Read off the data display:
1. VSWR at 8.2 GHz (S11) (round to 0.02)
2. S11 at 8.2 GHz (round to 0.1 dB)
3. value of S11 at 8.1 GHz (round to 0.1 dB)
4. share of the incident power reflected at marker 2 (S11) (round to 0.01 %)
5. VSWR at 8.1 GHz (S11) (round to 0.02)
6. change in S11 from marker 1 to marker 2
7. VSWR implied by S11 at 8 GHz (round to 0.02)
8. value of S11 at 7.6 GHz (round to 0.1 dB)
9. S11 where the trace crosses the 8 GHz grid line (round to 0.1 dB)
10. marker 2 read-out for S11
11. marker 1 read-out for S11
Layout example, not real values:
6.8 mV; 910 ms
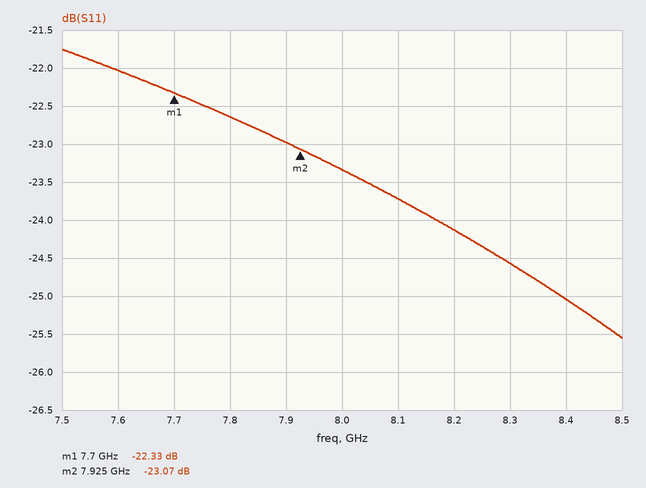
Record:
1.14; -24.1 dB; -23.7 dB; 0.49 %; 1.14; -0.74 dB; 1.14; -22.0 dB; -23.3 dB; -23.07 dB; -22.33 dB
